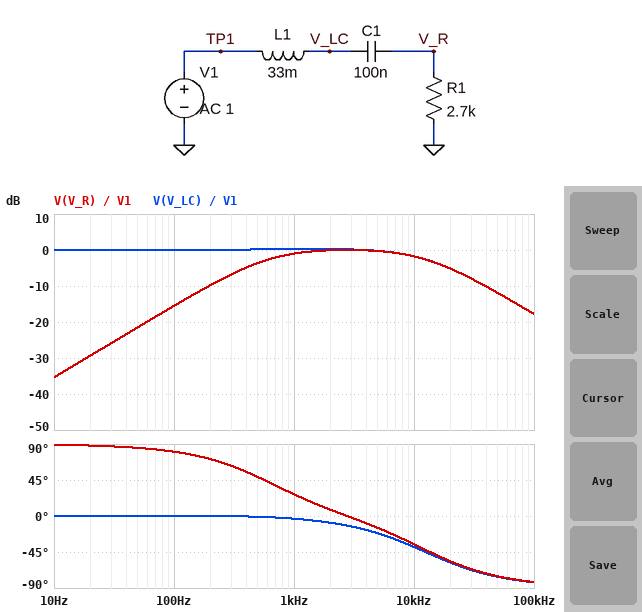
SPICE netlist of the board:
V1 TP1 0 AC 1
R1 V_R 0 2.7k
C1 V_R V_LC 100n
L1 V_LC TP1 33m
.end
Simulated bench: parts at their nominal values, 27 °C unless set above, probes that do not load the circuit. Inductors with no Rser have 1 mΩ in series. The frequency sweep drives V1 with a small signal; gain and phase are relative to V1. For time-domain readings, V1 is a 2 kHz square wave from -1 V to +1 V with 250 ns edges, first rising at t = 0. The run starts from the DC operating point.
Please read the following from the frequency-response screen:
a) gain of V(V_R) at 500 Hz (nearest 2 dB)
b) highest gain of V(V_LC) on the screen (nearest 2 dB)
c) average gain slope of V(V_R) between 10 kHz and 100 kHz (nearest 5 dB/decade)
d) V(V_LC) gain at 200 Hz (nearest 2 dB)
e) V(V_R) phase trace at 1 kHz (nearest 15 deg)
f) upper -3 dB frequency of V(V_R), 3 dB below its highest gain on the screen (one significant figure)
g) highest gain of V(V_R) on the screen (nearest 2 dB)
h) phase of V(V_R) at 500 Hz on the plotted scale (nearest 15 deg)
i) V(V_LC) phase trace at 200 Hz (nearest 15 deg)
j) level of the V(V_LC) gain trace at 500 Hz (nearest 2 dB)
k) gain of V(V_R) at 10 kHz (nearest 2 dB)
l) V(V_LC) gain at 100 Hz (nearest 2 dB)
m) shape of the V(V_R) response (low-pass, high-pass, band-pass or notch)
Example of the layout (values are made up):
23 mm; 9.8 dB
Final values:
-4 dB; 0 dB; -15 dB/decade; 0 dB; 30 deg; 10 kHz; 0 dB; 45 deg; 0 deg; 0 dB; -2 dB; 0 dB; band-pass
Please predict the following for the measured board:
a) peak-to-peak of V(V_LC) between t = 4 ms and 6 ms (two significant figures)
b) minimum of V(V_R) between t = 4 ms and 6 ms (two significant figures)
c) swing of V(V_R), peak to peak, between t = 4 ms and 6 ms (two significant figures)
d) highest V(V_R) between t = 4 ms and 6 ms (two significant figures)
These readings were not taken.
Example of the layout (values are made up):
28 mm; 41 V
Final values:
2.1 V; -1.3 V; 2.6 V; 1.3 V
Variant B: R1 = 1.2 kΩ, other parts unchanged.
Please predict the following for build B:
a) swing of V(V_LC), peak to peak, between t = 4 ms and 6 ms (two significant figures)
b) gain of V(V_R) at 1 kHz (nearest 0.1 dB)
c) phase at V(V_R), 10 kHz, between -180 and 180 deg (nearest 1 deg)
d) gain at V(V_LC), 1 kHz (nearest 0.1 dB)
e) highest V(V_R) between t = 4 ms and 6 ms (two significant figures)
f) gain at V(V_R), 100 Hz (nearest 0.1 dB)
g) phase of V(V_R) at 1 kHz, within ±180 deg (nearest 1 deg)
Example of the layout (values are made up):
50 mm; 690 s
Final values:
2.5 V; -3.7 dB; -58 deg; 0.7 dB; 1.4 V; -22.5 dB; 49 deg
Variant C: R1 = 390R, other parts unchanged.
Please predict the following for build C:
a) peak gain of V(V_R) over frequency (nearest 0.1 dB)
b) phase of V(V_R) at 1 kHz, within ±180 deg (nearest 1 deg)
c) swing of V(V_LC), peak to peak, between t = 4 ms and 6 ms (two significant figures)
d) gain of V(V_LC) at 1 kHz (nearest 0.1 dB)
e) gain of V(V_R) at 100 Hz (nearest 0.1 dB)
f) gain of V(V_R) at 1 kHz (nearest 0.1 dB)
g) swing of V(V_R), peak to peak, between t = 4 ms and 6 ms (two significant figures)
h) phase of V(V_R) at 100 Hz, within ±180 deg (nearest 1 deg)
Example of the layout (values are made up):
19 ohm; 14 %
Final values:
0 dB; 74 deg; 4.0 V; 1.1 dB; -32.2 dB; -11.3 dB; 2.1 V; 89 deg
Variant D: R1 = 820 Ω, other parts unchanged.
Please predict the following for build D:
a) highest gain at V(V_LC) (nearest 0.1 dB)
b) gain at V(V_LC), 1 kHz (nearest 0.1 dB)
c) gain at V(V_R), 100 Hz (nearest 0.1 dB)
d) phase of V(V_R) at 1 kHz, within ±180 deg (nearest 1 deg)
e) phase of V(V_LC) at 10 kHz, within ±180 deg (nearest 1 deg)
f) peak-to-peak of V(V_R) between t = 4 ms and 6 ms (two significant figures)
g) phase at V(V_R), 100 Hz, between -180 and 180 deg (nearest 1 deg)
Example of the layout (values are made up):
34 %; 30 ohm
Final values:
2.1 dB; 0.9 dB; -25.8 dB; 59 deg; -78 deg; 2.7 V; 87 deg
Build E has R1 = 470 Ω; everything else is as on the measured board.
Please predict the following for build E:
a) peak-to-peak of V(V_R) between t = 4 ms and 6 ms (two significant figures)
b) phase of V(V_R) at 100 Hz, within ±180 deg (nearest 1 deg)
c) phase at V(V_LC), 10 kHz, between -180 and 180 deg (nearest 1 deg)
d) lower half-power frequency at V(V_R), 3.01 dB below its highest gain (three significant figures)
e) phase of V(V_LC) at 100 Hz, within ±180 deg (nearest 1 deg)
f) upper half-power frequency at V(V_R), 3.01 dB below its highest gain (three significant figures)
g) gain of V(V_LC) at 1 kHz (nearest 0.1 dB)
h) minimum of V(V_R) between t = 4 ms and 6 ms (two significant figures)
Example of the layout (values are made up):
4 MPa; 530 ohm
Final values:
2.3 V; 88 deg; -95 deg; 1.86 kHz; 0 deg; 4.13 kHz; 1.1 dB; -1.2 V
